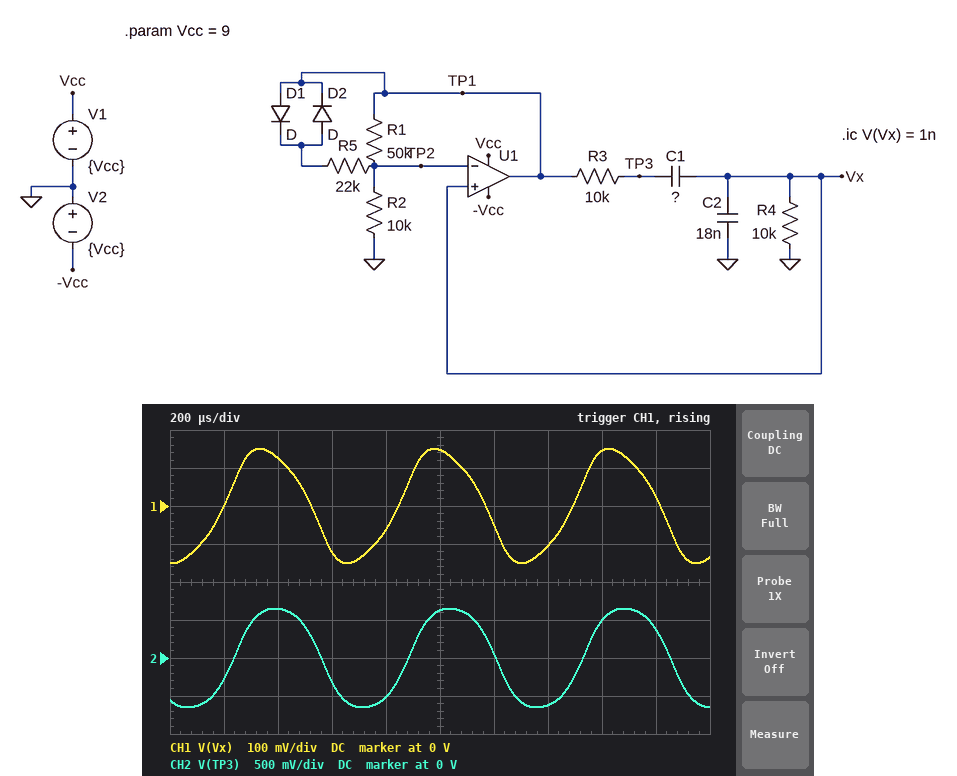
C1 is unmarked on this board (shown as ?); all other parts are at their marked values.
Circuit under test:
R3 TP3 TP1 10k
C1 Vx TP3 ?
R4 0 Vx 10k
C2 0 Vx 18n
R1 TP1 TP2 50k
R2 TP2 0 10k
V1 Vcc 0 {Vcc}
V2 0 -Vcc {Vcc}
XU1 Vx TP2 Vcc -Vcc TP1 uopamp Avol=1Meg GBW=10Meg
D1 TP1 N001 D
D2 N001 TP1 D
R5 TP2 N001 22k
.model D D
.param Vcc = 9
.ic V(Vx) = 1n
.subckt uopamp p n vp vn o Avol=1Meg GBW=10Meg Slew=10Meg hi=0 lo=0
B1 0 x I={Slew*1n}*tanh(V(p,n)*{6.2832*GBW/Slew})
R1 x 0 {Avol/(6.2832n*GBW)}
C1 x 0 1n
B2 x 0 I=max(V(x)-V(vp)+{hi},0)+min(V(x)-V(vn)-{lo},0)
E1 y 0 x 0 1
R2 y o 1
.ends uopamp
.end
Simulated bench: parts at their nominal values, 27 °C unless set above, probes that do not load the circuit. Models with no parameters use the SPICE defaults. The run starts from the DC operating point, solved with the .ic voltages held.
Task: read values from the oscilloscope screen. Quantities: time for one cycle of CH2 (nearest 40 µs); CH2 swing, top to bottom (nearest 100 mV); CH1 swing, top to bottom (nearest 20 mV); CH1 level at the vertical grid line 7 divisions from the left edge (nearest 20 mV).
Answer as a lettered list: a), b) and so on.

a) 640 µs
b) 1.3 V
c) 300 mV
d) -100 mV
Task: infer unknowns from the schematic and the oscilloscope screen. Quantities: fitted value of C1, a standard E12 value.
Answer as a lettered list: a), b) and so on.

a) 5.6 nF
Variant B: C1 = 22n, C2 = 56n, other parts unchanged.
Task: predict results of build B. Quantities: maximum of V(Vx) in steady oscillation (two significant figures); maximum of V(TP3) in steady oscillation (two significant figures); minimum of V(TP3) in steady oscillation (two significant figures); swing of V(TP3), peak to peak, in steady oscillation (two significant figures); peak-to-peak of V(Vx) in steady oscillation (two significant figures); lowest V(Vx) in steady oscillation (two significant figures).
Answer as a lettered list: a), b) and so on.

a) 220 mV
b) 790 mV
c) -790 mV
d) 1.6 V
e) 440 mV
f) -220 mV
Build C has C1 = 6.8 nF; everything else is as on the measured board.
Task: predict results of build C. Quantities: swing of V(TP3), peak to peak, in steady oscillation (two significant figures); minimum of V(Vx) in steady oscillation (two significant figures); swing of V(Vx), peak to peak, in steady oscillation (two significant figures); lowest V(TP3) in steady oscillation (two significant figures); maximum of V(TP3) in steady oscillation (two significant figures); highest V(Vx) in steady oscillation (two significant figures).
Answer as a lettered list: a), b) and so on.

a) 1.5 V
b) -210 mV
c) 410 mV
d) -770 mV
e) 770 mV
f) 210 mV
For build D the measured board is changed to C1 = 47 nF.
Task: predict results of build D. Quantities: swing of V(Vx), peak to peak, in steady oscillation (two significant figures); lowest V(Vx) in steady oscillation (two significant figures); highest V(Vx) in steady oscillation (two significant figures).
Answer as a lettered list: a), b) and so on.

a) 8.6 V
b) -4.3 V
c) 4.3 V
